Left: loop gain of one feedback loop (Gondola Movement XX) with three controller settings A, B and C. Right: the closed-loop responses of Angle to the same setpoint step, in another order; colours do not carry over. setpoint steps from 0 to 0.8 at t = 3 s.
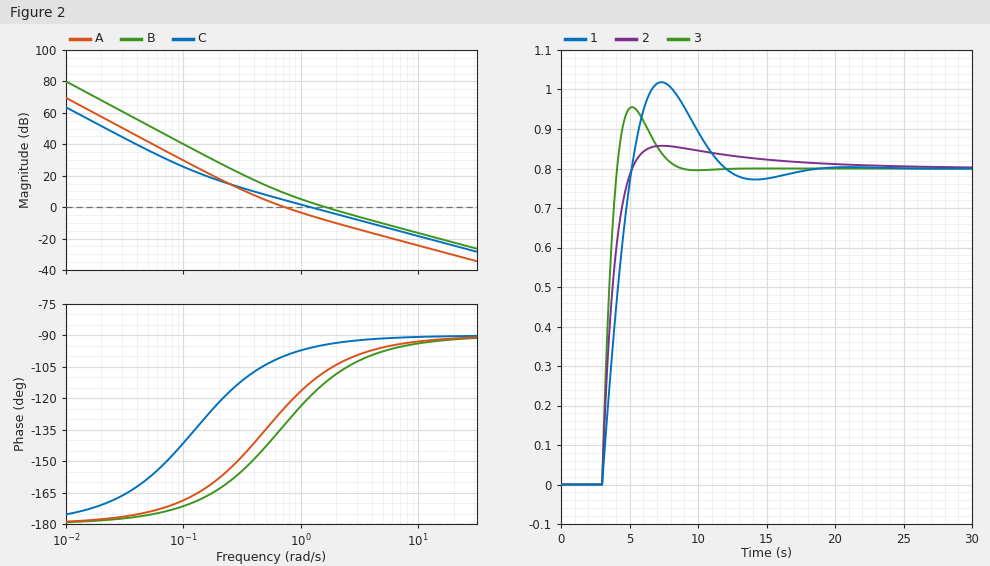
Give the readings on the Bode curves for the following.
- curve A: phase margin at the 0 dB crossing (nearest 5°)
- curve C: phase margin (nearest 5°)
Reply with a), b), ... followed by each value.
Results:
a) 55°
b) 85°
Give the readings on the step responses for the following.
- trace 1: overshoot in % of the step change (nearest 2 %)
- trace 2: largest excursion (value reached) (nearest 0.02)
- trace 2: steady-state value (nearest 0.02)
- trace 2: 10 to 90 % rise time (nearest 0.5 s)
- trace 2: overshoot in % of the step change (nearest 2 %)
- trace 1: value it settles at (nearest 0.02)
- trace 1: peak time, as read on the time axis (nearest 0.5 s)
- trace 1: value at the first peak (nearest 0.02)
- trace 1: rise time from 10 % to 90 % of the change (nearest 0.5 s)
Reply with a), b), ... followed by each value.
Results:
a) 28 %
b) 0.86
c) 0.80
d) 1.5 s
e) 8 %
f) 0.80
g) 7.5 s
h) 1.02
i) 1.5 s
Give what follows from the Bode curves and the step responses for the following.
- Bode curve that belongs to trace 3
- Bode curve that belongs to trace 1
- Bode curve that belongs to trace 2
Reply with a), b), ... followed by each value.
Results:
a) B
b) A
c) C
